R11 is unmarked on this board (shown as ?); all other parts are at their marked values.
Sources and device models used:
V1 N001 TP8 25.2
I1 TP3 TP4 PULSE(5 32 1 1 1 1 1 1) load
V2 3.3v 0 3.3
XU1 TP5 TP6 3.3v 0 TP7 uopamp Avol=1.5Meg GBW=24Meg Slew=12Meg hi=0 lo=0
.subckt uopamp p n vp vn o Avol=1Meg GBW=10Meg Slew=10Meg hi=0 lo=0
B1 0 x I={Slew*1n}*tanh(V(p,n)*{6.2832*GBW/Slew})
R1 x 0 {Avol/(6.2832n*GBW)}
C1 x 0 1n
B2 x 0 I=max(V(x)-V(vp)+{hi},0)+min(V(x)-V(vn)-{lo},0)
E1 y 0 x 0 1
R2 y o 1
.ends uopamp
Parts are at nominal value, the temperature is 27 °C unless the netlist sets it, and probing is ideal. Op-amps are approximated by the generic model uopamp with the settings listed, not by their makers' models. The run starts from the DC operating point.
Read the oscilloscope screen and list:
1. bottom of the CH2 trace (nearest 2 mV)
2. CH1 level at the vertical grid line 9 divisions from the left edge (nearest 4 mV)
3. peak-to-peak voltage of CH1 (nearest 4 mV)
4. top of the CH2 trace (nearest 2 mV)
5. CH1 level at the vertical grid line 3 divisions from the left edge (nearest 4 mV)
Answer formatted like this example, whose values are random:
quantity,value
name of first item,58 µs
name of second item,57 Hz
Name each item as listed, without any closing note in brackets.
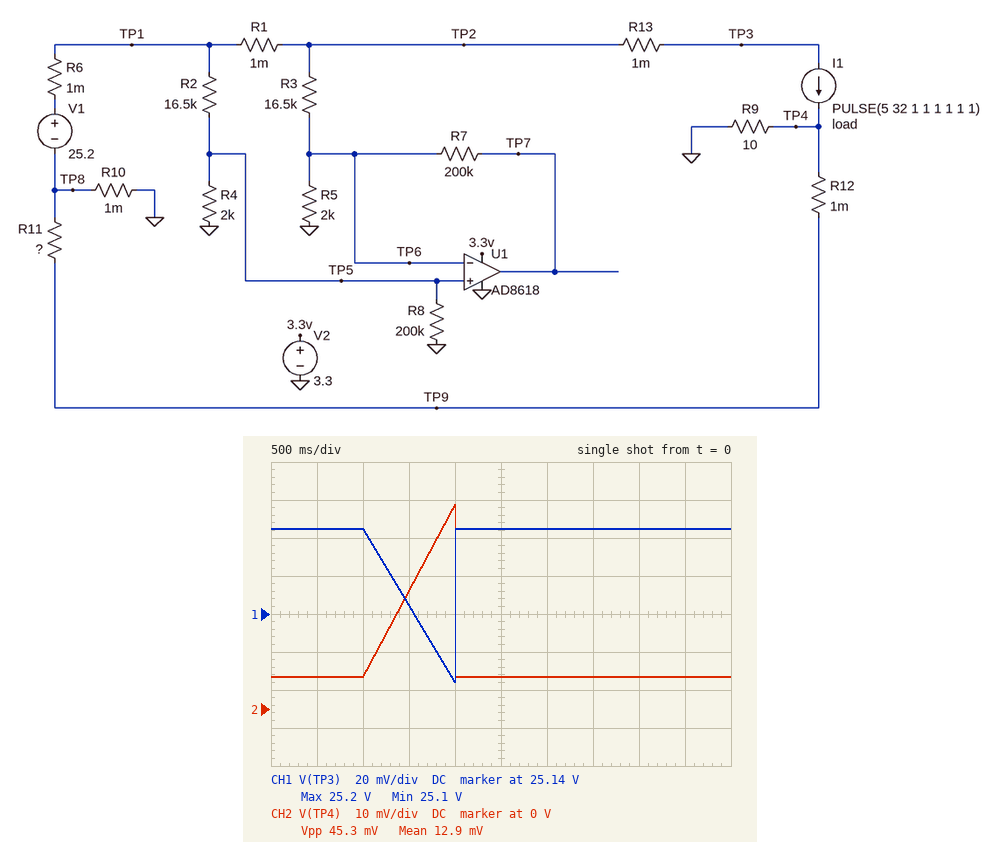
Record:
quantity,value
bottom of the CH2 trace,8 mV
CH1 level at the vertical grid line 9 divisions from the left edge,25.184 V
peak-to-peak voltage of CH1,80 mV
top of the CH2 trace,54 mV
CH1 level at the vertical grid line 3 divisions from the left edge,25.144 V
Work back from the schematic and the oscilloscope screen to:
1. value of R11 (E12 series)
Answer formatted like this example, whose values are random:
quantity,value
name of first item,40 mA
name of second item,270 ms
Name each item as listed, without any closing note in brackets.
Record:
quantity,value
value of R11,680 µΩ
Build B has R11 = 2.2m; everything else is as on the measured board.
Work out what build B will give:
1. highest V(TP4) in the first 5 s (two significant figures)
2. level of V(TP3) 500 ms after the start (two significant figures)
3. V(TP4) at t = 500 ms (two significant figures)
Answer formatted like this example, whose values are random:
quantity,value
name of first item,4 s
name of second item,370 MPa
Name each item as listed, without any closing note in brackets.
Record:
quantity,value
highest V(TP4) in the first 5 s,100 mV
level of V(TP3) 500 ms after the start,25 V
V(TP4) at t = 500 ms,16 mV
